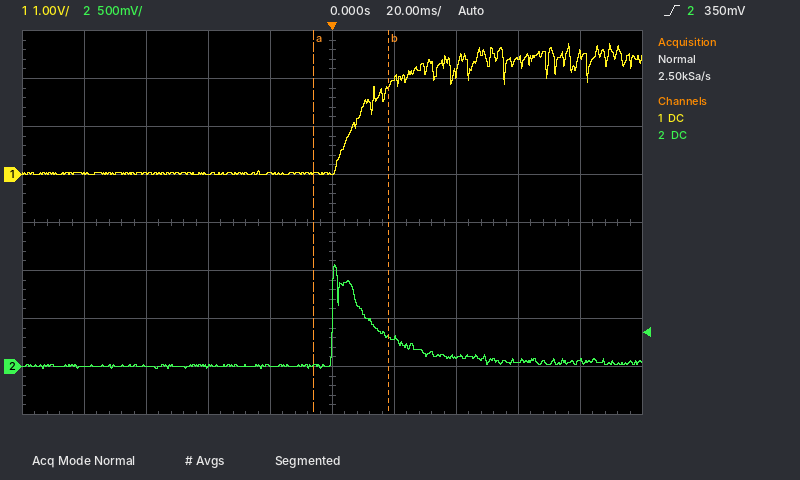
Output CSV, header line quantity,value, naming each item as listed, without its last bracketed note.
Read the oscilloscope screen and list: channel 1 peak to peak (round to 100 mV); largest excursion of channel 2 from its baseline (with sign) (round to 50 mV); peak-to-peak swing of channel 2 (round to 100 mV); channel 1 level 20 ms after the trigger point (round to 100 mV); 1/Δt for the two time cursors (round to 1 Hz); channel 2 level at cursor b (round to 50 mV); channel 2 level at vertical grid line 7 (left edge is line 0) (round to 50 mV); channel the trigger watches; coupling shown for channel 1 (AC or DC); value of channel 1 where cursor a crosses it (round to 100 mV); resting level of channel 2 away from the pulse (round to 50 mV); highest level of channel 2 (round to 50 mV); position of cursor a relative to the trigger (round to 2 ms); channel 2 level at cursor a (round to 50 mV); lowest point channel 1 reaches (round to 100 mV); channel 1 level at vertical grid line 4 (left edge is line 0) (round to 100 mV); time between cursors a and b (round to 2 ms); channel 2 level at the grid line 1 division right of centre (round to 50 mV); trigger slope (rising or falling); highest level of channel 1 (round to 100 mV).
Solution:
quantity,value
channel 1 peak to peak,2.7 V
largest excursion of channel 2 from its baseline (with sign),+1.05 V
peak-to-peak swing of channel 2,1.10 V
channel 1 level 20 ms after the trigger point,2.0 V
1/Δt for the two time cursors,42 Hz
channel 2 level at cursor b,300 mV
channel 2 level at vertical grid line 7 (left edge is line 0),100 mV
channel the trigger watches,channel 2
coupling shown for channel 1,DC
value of channel 1 where cursor a crosses it,0.0 V
resting level of channel 2 away from the pulse,0 mV
highest level of channel 2,1.05 V
position of cursor a relative to the trigger,-6 ms
channel 2 level at cursor a,0 mV
lowest point channel 1 reaches,0.0 V
channel 1 level at vertical grid line 4 (left edge is line 0),0.0 V
time between cursors a and b,24 ms
channel 2 level at the grid line 1 division right of centre,300 mV
trigger slope,rising
highest level of channel 1,2.7 V
